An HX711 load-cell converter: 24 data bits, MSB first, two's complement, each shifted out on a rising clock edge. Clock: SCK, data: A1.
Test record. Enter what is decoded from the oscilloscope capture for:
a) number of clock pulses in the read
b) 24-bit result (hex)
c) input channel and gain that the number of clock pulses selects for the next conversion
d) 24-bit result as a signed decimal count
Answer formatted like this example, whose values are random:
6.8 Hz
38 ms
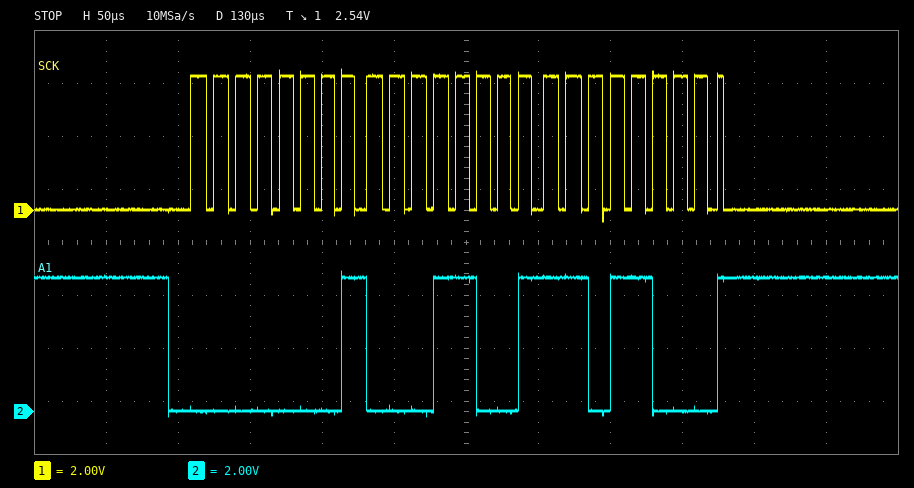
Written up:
25
0x0119D8
channel A, gain 128
72152
